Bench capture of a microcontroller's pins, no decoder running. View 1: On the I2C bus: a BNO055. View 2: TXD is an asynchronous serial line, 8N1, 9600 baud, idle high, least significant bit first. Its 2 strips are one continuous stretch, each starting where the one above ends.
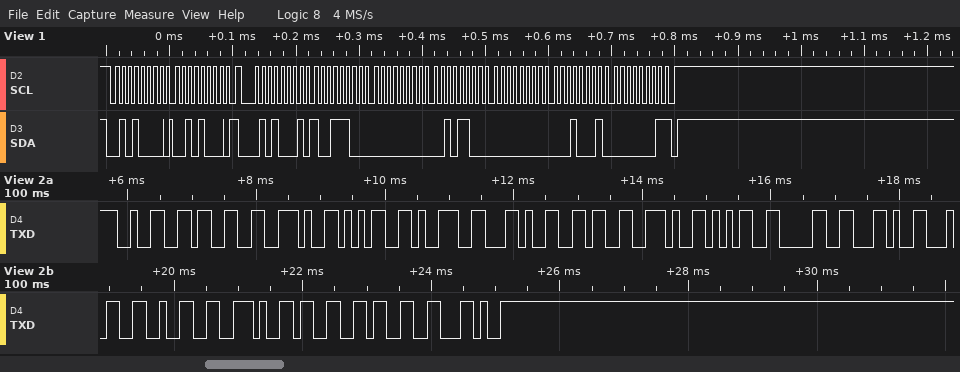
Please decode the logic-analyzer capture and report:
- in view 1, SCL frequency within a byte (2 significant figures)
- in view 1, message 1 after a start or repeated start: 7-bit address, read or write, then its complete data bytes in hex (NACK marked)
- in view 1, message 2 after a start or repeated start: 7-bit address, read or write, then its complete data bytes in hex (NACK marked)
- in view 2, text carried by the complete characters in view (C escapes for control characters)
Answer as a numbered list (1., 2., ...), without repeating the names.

1. 100 kHz
2. 0x28 write: 28
3. 0x28 read: 9C 00 2C 00 11 01 NACK
4. "23.59,6.50,42.33,"
